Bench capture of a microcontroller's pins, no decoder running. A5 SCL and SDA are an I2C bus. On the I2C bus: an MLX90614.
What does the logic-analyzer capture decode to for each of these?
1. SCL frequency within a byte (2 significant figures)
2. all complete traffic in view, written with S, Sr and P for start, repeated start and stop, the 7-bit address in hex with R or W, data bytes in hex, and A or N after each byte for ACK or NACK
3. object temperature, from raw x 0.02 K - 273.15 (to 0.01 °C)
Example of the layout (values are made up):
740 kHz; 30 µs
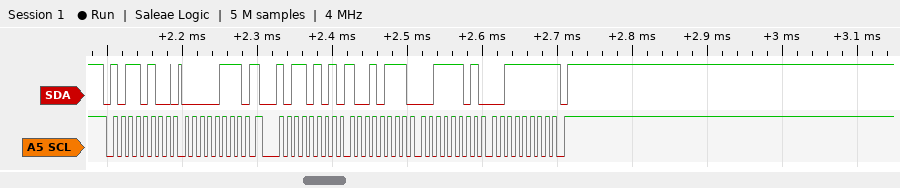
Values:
100 kHz; S 5AW A 07 A Sr 5AR A 97 A 3D A 3F N P; 42.19 °C
